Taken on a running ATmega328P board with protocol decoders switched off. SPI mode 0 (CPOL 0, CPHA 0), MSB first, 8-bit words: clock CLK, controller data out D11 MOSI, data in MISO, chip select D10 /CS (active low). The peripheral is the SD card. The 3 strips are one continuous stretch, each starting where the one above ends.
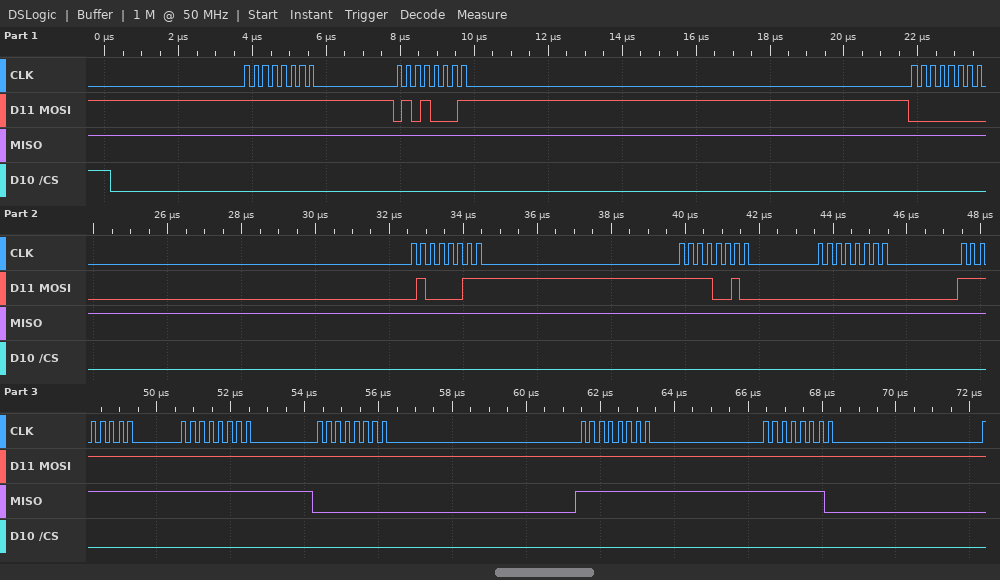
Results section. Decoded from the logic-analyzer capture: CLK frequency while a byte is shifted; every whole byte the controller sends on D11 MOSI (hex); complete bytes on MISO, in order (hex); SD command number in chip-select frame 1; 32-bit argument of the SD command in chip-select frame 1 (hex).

4 MHz
0xFF 0x51 0x00 0x43 0xF2 0x00 0xFF 0xFF 0xFF 0xFF 0xFF
0xFF 0xFF 0xFF 0xFF 0xFF 0xFF 0xFF 0xFF 0x00 0xFF 0xFE
CMD17
0x0043F200
